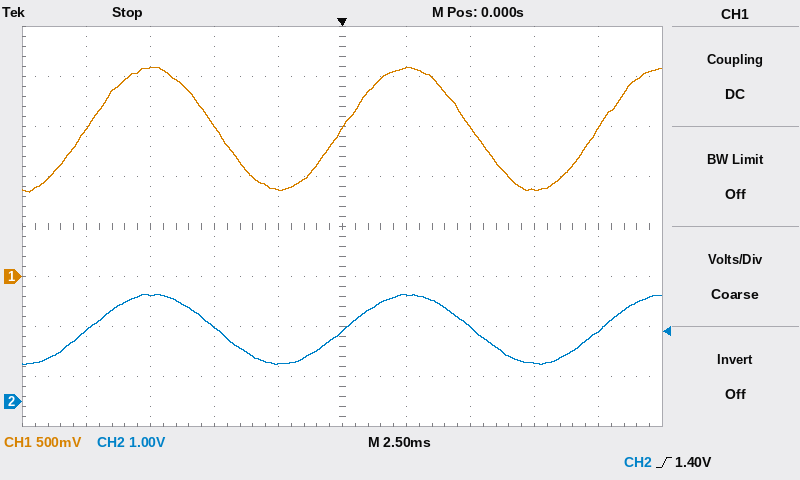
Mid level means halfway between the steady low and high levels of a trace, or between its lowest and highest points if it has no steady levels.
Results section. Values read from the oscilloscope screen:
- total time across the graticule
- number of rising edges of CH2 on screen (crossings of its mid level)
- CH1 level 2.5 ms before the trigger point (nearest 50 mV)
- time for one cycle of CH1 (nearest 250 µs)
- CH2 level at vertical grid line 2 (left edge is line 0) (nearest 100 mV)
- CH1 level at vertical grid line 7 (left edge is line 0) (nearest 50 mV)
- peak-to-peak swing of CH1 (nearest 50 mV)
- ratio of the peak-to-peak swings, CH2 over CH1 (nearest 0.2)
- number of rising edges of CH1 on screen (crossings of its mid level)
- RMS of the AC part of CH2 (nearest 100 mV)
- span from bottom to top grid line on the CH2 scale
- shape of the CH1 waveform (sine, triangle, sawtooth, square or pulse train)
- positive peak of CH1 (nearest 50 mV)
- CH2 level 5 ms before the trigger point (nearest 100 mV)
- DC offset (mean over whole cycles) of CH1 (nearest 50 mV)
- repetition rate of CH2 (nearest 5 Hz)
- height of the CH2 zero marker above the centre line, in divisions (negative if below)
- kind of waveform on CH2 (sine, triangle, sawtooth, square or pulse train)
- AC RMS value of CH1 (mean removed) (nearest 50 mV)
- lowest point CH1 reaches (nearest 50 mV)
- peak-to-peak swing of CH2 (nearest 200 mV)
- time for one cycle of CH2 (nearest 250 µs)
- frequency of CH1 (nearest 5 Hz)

25 ms
3
850 mV
10.00 ms
2.1 V
1.50 V
1.25 V
1.2
3
500 mV
8 V
sine
2.10 V
1.5 V
1.50 V
100 Hz
-3.5 div
sine
450 mV
850 mV
1.4 V
10.00 ms
100 Hz
